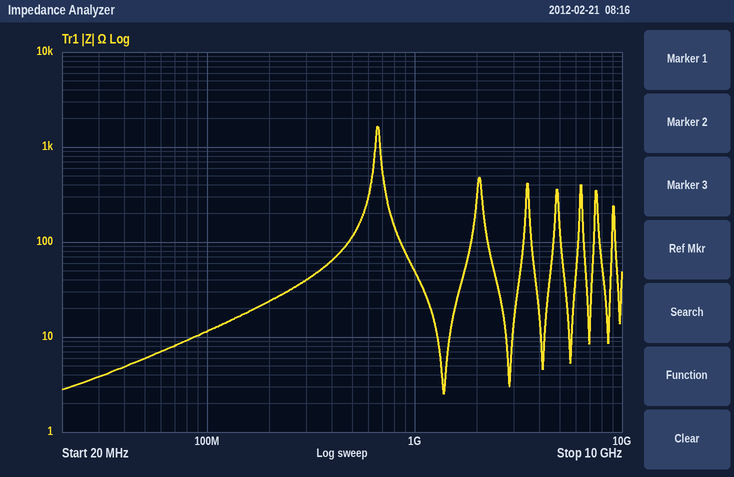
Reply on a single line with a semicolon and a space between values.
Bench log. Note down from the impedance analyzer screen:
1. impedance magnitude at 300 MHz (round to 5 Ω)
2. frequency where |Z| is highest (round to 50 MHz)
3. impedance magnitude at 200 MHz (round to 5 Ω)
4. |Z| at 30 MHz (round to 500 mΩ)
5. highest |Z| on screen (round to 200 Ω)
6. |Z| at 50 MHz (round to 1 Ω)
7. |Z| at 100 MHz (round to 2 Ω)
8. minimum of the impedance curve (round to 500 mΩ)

40 Ω; 650 MHz; 25 Ω; 4.0 Ω; 1.6 kΩ; 6 Ω; 12 Ω; 2.5 Ω
